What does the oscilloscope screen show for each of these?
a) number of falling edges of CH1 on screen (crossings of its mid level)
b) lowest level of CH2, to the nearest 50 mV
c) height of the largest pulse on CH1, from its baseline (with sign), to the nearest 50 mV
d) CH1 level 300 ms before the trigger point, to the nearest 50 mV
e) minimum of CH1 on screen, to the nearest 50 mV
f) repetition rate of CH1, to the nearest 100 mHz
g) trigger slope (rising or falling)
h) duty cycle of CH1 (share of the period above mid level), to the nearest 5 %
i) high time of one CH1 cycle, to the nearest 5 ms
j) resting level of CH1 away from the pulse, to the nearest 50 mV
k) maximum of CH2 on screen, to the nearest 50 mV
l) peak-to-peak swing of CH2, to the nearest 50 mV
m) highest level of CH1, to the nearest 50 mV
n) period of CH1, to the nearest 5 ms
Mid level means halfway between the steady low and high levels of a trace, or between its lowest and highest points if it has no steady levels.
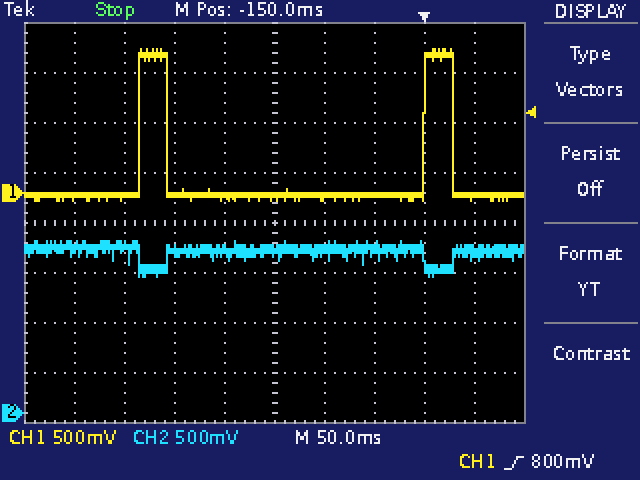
2
1.35 V
+1.45 V
-50 mV
-100 mV
3.5 Hz
rising
10 %
30 ms
0 mV
1.70 V
350 mV
1.45 V
285 ms
